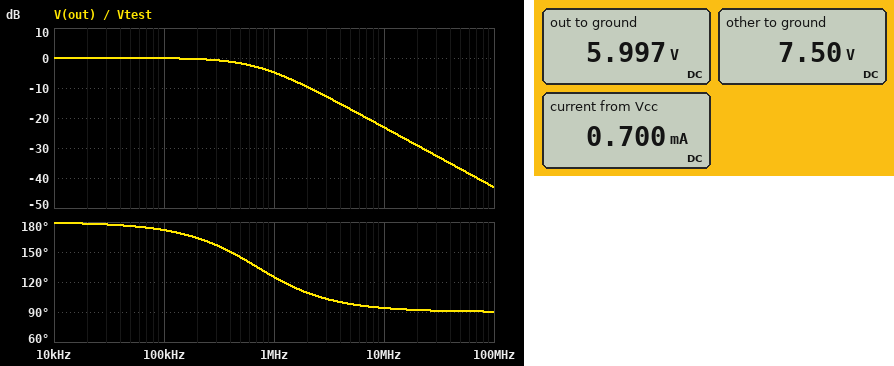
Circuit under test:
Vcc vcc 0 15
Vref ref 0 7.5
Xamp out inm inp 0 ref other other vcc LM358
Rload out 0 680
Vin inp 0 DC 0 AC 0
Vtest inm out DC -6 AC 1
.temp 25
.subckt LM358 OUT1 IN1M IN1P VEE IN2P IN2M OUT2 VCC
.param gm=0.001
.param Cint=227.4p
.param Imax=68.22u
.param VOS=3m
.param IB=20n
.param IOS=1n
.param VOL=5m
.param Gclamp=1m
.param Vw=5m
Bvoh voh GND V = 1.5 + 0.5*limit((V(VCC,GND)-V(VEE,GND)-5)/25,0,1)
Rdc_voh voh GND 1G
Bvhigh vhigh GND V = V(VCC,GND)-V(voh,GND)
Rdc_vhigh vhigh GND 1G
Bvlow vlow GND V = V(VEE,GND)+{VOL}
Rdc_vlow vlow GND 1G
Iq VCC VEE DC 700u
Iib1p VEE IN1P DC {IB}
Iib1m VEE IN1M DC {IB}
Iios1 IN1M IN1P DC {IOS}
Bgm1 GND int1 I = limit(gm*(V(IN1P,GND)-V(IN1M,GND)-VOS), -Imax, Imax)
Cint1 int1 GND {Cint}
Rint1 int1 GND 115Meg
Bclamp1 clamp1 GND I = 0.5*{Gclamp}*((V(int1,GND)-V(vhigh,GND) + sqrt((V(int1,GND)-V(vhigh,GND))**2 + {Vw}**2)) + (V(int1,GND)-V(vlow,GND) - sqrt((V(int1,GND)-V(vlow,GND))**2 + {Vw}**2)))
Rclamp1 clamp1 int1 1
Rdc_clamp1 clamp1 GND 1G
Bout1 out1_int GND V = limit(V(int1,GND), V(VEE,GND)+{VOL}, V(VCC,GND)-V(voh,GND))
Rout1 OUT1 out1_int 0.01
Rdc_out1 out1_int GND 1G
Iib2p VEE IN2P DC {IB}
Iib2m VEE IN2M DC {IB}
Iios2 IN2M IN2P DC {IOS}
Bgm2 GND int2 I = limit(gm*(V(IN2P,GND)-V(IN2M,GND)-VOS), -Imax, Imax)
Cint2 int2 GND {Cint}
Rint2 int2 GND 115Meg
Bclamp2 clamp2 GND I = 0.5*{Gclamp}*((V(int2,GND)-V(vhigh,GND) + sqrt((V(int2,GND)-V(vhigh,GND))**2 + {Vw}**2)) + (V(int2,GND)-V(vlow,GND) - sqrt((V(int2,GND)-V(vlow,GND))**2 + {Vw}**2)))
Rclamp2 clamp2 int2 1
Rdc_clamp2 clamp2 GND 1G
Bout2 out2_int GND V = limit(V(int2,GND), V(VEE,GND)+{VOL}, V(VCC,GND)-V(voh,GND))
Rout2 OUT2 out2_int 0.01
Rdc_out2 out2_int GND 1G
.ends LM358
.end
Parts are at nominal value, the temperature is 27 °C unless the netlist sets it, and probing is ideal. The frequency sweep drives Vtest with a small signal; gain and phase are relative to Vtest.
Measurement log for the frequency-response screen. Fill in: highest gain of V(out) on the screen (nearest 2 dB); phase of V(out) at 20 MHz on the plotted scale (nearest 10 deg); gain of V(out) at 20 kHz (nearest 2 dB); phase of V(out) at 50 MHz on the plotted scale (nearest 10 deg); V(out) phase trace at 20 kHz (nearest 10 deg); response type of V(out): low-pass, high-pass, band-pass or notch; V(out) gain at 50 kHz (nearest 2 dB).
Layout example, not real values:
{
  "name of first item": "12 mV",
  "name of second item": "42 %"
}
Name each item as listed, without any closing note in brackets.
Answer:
{
  "highest gain of V(out) on the screen": "0 dB",
  "phase of V(out) at 20 MHz on the plotted scale": "90 deg",
  "gain of V(out) at 20 kHz": "0 dB",
  "phase of V(out) at 50 MHz on the plotted scale": "90 deg",
  "V(out) phase trace at 20 kHz": "180 deg",
  "response type of V(out): low-pass, high-pass, band-pass or notch": "low-pass",
  "V(out) gain at 50 kHz": "0 dB"
}
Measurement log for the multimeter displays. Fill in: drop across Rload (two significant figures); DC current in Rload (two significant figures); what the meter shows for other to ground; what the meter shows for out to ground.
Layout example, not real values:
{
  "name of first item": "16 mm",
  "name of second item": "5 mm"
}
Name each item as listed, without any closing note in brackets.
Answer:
{
  "drop across Rload": "6.0 V",
  "DC current in Rload": "8.8 mA",
  "what the meter shows for other to ground": "7.50 V",
  "what the meter shows for out to ground": "5.997 V"
}
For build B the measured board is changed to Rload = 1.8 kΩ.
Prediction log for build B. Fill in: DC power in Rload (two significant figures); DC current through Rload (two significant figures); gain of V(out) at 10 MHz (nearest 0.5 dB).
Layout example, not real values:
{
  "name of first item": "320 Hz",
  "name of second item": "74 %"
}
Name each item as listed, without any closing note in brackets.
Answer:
{
  "DC power in Rload": "20 mW",
  "DC current through Rload": "3.3 mA",
  "gain of V(out) at 10 MHz": "-23.0 dB"
}
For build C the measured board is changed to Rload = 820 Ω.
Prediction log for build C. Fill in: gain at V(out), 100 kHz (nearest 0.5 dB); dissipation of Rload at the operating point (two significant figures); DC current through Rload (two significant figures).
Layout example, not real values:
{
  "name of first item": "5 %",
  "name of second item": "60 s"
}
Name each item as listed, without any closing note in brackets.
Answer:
{
  "gain at V(out), 100 kHz": "0 dB",
  "dissipation of Rload at the operating point": "44 mW",
  "DC current through Rload": "7.3 mA"
}
